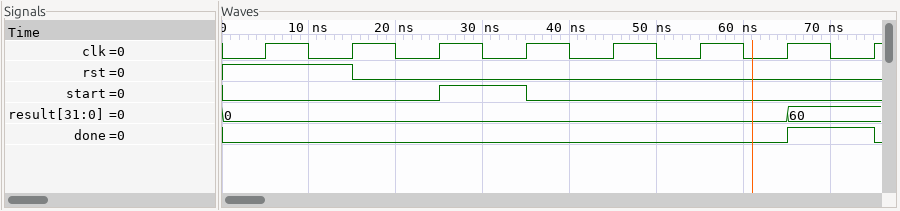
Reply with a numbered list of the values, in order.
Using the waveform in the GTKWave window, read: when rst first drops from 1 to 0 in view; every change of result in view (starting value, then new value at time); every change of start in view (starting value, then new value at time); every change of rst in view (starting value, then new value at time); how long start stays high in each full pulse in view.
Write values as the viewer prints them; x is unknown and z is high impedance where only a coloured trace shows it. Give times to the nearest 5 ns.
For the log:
1. 15 ns
2. 0, 60 at 65 ns
3. 0, 1 at 25 ns, 0 at 35 ns
4. 1, 0 at 15 ns
5. 10 ns
